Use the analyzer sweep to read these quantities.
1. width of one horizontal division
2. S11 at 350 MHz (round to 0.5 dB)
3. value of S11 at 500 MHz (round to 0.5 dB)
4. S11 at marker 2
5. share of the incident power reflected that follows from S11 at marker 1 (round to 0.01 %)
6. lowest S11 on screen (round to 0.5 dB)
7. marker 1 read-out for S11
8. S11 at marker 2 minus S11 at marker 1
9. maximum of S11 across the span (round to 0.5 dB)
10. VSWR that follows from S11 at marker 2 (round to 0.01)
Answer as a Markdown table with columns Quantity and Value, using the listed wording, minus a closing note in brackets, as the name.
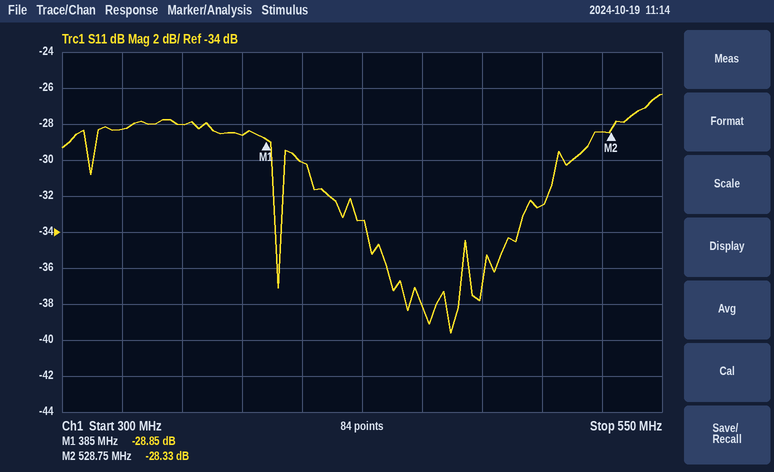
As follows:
| Quantity | Value |
|---|---|
| width of one horizontal division | 25 MHz |
| S11 at 350 MHz | -28.0 dB |
| value of S11 at 500 MHz | -32.5 dB |
| S11 at marker 2 | -28.33 dB |
| share of the incident power reflected that follows from S11 at marker 1 | 0.13 % |
| lowest S11 on screen | -39.5 dB |
| marker 1 read-out for S11 | -28.85 dB |
| S11 at marker 2 minus S11 at marker 1 | 0.52 dB |
| maximum of S11 across the span | -26.5 dB |
| VSWR that follows from S11 at marker 2 | 1.08 |
